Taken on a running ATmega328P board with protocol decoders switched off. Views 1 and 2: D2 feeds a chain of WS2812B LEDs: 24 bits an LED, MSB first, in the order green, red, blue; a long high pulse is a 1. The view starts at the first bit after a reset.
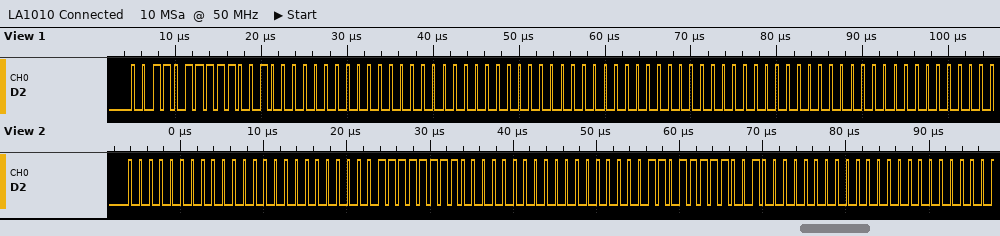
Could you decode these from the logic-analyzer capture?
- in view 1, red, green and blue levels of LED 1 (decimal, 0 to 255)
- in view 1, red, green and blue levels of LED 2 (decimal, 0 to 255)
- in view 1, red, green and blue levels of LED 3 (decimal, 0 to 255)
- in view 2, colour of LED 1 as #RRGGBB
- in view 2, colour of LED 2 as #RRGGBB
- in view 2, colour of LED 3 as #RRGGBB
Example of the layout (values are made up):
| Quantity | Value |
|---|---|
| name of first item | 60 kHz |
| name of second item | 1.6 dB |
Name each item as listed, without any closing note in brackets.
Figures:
| Quantity | Value |
|---|---|
| in view 1, red, green and blue levels of LED 1 | 200, 55, 0 |
| in view 1, red, green and blue levels of LED 2 | 0, 0, 0 |
| in view 1, red, green and blue levels of LED 3 | 0, 0, 0 |
| in view 2, colour of LED 1 as #RRGGBB | #000000 |
| in view 2, colour of LED 2 as #RRGGBB | #00FF00 |
| in view 2, colour of LED 3 as #RRGGBB | #C83700 |
